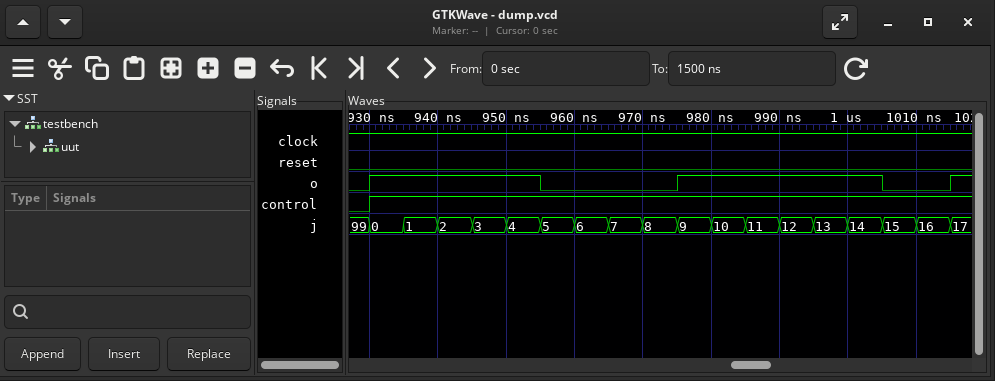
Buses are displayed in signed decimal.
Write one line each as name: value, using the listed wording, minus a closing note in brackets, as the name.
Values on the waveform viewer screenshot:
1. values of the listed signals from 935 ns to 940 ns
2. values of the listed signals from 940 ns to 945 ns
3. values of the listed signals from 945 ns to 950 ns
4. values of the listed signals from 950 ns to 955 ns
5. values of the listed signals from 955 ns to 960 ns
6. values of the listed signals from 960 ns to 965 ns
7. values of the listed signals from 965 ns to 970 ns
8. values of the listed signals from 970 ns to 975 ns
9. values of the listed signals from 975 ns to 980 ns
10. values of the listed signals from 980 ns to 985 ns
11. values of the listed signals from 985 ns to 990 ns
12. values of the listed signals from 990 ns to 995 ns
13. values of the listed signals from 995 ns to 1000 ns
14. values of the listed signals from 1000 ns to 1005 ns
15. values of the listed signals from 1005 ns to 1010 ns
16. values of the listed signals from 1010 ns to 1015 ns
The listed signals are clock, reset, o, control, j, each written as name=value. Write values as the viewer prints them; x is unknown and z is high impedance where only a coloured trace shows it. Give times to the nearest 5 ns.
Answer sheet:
values of the listed signals from 935 ns to 940 ns: clock=1, reset=0, o=1, control=1, j=1
values of the listed signals from 940 ns to 945 ns: clock=1, reset=0, o=1, control=1, j=2
values of the listed signals from 945 ns to 950 ns: clock=1, reset=0, o=1, control=1, j=3
values of the listed signals from 950 ns to 955 ns: clock=1, reset=0, o=1, control=1, j=4
values of the listed signals from 955 ns to 960 ns: clock=1, reset=0, o=0, control=1, j=5
values of the listed signals from 960 ns to 965 ns: clock=1, reset=0, o=0, control=1, j=6
values of the listed signals from 965 ns to 970 ns: clock=1, reset=0, o=0, control=1, j=7
values of the listed signals from 970 ns to 975 ns: clock=1, reset=0, o=0, control=1, j=8
values of the listed signals from 975 ns to 980 ns: clock=1, reset=0, o=1, control=1, j=9
values of the listed signals from 980 ns to 985 ns: clock=1, reset=0, o=1, control=1, j=10
values of the listed signals from 985 ns to 990 ns: clock=1, reset=0, o=1, control=1, j=11
values of the listed signals from 990 ns to 995 ns: clock=1, reset=0, o=1, control=1, j=12
values of the listed signals from 995 ns to 1000 ns: clock=1, reset=0, o=1, control=1, j=13
values of the listed signals from 1000 ns to 1005 ns: clock=1, reset=0, o=1, control=1, j=14
values of the listed signals from 1005 ns to 1010 ns: clock=1, reset=0, o=0, control=1, j=15
values of the listed signals from 1010 ns to 1015 ns: clock=1, reset=0, o=0, control=1, j=16
